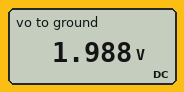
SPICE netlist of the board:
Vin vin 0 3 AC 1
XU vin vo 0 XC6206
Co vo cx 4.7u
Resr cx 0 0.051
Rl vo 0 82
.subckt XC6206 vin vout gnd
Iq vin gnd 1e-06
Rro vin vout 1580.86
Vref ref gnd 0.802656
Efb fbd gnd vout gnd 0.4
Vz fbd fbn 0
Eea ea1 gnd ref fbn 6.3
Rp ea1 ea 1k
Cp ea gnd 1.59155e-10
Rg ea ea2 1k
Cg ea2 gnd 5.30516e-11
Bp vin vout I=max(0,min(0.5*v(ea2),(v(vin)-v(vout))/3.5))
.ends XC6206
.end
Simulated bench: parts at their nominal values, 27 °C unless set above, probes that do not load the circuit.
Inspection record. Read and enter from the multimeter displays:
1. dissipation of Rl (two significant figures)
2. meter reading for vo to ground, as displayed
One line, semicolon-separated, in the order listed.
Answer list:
48 mW; 1.988 V
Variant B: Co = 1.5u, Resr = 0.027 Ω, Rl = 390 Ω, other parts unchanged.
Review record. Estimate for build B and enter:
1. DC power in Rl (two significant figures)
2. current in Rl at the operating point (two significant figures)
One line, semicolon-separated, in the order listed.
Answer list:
10 mW; 5.1 mA
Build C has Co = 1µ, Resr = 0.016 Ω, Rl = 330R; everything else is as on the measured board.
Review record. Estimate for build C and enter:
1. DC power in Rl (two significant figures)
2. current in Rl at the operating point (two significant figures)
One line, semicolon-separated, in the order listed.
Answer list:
12 mW; 6.1 mA
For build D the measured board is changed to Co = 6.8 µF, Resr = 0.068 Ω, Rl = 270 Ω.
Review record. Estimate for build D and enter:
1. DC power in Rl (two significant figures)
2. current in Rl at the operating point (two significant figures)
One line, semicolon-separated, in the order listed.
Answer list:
15 mW; 7.4 mA
